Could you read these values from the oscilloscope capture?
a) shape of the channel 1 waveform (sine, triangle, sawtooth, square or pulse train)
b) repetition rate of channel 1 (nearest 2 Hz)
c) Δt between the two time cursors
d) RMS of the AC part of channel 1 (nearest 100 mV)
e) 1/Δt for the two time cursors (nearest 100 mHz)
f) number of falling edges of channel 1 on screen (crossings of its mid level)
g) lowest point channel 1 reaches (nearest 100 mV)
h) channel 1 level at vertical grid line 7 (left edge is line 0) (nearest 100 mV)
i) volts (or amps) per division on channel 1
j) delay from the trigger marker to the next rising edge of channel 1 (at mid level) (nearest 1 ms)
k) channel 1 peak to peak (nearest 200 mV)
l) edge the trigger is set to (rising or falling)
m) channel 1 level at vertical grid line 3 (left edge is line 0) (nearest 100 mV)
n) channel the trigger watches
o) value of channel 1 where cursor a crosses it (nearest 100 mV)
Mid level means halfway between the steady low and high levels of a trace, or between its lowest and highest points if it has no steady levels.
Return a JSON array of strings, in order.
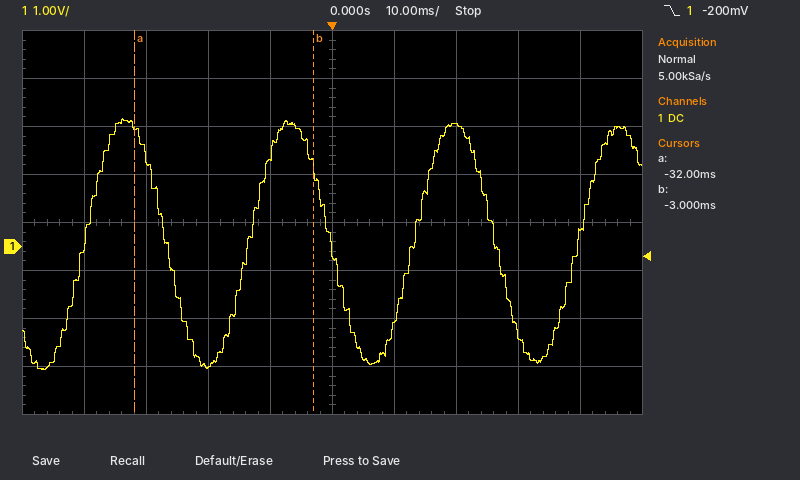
["sine", "38 Hz", "29 ms", "1.8 V", "34.5 Hz", "3", "-2.6 V", "2.5 V", "1 V", "13 ms", "5.2 V", "falling", "-2.5 V", "channel 1", "2.5 V"]
